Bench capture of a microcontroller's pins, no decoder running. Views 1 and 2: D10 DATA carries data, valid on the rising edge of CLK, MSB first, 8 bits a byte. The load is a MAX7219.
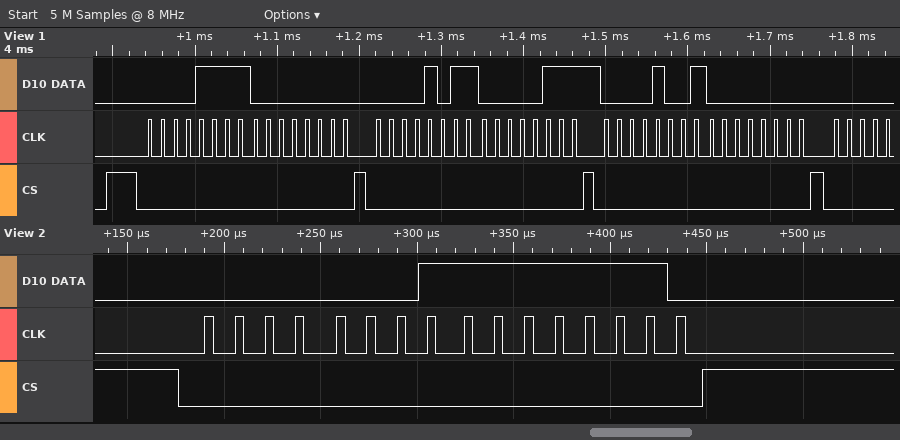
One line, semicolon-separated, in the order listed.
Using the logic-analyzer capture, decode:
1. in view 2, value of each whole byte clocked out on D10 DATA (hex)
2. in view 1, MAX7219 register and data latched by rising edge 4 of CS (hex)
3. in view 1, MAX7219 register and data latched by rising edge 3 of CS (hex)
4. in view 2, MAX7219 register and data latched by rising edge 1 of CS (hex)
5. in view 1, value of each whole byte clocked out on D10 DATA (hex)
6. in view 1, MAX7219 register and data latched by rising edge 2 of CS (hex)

0x01 0xFE; register 0x9, data 0x00; register 0xB, data 0x07; register 0x1, data 0xFE; 0F 00 0B 07 09 00; register 0xF, data 0x00
